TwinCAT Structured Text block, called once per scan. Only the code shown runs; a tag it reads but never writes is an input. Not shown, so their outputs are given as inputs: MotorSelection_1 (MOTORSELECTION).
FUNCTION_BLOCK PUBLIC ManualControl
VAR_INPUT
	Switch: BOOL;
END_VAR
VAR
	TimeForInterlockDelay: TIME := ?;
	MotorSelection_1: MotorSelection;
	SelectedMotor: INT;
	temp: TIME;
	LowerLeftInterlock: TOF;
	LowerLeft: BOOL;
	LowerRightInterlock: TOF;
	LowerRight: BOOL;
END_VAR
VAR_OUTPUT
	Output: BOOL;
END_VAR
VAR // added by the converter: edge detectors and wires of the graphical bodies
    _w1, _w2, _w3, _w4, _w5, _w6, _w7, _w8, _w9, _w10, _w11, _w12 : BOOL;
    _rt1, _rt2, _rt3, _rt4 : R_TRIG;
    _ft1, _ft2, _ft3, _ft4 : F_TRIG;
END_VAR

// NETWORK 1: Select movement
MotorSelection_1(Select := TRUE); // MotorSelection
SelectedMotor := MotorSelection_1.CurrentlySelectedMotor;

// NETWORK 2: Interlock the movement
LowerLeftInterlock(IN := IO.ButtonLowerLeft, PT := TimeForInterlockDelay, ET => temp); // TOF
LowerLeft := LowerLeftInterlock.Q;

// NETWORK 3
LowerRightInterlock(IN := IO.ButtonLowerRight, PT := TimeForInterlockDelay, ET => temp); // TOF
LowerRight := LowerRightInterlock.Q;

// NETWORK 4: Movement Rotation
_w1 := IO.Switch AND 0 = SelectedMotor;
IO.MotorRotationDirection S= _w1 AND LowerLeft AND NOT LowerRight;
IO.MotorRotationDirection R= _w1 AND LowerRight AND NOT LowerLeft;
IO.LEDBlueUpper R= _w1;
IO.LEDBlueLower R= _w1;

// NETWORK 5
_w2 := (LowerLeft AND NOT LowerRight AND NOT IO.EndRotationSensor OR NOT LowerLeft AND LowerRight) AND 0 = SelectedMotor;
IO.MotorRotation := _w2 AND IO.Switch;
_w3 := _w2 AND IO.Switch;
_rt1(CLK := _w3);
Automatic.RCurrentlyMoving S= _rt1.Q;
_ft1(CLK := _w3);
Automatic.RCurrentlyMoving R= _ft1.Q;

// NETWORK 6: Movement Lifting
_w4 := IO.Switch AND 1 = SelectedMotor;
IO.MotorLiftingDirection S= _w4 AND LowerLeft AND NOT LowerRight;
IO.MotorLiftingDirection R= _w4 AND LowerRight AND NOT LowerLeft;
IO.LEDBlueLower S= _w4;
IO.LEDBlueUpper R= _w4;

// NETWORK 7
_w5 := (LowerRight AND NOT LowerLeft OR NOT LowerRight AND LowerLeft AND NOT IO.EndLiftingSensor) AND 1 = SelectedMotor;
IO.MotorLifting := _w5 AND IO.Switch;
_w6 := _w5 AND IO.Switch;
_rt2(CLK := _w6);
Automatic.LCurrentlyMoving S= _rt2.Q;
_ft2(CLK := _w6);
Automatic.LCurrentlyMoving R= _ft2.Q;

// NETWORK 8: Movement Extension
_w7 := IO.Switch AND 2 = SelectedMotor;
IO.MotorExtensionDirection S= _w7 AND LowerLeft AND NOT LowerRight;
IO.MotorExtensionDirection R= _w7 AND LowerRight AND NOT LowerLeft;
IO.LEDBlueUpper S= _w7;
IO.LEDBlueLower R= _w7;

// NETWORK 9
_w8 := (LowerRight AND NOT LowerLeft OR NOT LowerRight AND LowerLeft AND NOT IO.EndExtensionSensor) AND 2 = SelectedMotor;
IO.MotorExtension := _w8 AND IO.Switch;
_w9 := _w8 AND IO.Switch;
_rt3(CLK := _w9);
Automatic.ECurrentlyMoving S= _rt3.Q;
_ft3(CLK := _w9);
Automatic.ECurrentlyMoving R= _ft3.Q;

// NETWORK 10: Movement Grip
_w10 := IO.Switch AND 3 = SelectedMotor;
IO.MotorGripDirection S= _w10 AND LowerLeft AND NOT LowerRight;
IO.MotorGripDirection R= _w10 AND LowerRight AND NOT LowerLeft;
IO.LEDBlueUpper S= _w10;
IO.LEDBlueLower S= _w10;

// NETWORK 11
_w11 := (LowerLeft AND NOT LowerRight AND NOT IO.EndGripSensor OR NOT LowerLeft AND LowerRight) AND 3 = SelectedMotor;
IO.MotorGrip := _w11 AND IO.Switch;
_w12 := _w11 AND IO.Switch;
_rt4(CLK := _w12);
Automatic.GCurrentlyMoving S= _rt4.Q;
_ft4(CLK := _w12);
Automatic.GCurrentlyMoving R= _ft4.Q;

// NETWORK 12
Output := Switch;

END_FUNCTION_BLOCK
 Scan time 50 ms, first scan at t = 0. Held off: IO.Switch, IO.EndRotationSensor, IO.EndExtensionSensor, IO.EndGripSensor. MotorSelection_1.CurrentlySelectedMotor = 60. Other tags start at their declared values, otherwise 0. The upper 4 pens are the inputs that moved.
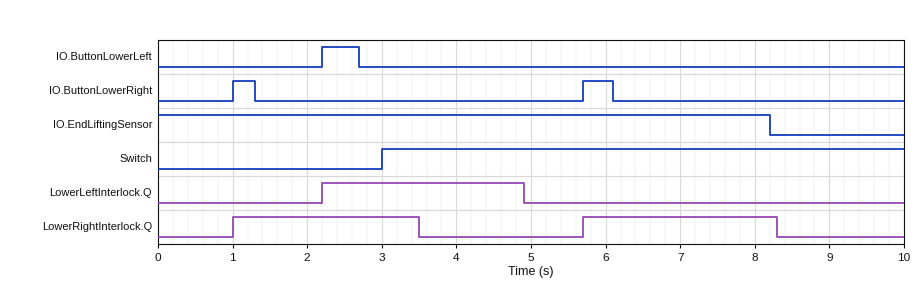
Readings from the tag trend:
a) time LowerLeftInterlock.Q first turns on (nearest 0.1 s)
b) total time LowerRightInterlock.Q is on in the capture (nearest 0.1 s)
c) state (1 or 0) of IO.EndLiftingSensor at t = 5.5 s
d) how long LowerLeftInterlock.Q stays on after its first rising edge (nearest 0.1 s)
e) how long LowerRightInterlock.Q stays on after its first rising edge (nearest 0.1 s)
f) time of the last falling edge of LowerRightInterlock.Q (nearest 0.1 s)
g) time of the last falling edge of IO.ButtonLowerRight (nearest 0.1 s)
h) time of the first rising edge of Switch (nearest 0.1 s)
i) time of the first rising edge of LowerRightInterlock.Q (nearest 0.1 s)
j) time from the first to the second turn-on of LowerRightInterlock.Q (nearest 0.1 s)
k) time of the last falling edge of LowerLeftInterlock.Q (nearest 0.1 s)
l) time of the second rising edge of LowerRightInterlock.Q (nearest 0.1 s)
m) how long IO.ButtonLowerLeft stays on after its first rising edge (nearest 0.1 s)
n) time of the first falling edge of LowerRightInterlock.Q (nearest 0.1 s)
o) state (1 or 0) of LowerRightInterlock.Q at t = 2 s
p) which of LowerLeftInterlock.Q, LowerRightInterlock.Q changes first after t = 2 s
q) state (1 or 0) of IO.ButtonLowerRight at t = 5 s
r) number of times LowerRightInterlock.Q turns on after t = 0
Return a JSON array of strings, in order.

["2.2 s", "5.1 s", "1", "2.7 s", "2.5 s", "8.3 s", "6.1 s", "3.0 s", "1.0 s", "4.7 s", "4.9 s", "5.7 s", "0.5 s", "3.5 s", "1", "LowerLeftInterlock.Q", "0", "2"]
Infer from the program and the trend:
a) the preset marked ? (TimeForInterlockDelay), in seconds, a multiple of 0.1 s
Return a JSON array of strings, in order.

["2.2 s"]
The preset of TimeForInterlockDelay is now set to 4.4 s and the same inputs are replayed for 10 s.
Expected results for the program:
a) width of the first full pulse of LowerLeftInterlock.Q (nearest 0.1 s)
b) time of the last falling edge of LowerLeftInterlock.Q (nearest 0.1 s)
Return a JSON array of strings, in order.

["4.9 s", "7.1 s"]
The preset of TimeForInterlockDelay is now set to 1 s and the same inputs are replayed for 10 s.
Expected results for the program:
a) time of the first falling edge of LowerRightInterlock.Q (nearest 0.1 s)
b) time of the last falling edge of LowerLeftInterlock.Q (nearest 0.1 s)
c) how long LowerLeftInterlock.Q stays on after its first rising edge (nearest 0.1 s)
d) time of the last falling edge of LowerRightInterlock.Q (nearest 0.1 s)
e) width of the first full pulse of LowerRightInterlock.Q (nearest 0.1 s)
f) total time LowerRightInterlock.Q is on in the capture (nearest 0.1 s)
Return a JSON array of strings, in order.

["2.3 s", "3.7 s", "1.5 s", "7.1 s", "1.3 s", "2.7 s"]
